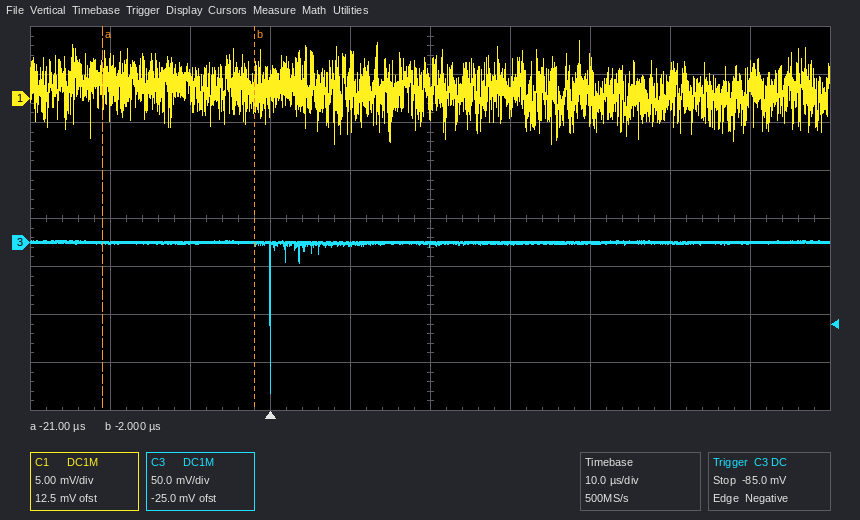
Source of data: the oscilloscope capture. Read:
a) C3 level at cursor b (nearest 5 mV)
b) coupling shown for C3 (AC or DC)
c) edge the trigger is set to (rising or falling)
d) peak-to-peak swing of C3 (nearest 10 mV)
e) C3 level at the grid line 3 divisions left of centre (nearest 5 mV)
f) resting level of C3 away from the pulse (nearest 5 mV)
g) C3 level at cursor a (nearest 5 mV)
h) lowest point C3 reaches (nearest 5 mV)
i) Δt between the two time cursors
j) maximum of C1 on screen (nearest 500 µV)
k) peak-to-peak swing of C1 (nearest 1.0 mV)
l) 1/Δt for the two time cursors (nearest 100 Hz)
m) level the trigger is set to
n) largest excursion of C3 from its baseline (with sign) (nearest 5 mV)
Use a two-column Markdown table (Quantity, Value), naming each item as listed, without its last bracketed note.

| Quantity | Value |
|---|---|
| C3 level at cursor b | 0 mV |
| coupling shown for C3 | DC |
| edge the trigger is set to | falling |
| peak-to-peak swing of C3 | 160 mV |
| C3 level at the grid line 3 divisions left of centre | 0 mV |
| resting level of C3 away from the pulse | 0 mV |
| C3 level at cursor a | 0 mV |
| lowest point C3 reaches | -155 mV |
| Δt between the two time cursors | 19 µs |
| maximum of C1 on screen | 6.0 mV |
| peak-to-peak swing of C1 | 11.0 mV |
| 1/Δt for the two time cursors | 52.6 kHz |
| level the trigger is set to | -85.0 mV |
| largest excursion of C3 from its baseline (with sign) | -155 mV |
